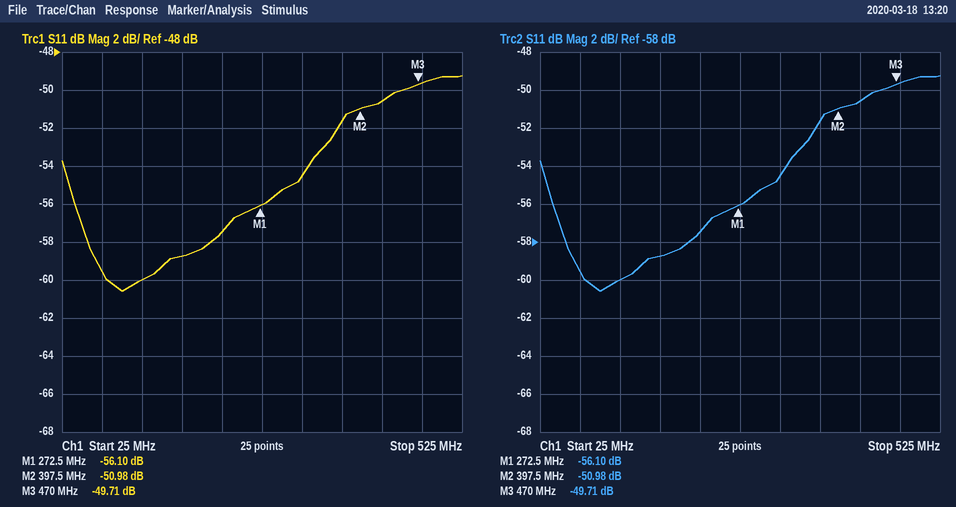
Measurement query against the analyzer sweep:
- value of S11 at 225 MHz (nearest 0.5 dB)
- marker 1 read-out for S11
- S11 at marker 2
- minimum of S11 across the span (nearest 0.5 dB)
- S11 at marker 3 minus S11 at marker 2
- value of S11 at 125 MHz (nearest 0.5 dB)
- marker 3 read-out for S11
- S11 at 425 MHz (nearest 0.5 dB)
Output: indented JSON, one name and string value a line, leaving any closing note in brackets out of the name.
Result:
{
  "value of S11 at 225 MHz": "-57.5 dB",
  "marker 1 read-out for S11": "-56.10 dB",
  "S11 at marker 2": "-50.98 dB",
  "minimum of S11 across the span": "-60.5 dB",
  "S11 at marker 3 minus S11 at marker 2": "1.27 dB",
  "value of S11 at 125 MHz": "-60.0 dB",
  "marker 3 read-out for S11": "-49.71 dB",
  "S11 at 425 MHz": "-50.5 dB"
}
